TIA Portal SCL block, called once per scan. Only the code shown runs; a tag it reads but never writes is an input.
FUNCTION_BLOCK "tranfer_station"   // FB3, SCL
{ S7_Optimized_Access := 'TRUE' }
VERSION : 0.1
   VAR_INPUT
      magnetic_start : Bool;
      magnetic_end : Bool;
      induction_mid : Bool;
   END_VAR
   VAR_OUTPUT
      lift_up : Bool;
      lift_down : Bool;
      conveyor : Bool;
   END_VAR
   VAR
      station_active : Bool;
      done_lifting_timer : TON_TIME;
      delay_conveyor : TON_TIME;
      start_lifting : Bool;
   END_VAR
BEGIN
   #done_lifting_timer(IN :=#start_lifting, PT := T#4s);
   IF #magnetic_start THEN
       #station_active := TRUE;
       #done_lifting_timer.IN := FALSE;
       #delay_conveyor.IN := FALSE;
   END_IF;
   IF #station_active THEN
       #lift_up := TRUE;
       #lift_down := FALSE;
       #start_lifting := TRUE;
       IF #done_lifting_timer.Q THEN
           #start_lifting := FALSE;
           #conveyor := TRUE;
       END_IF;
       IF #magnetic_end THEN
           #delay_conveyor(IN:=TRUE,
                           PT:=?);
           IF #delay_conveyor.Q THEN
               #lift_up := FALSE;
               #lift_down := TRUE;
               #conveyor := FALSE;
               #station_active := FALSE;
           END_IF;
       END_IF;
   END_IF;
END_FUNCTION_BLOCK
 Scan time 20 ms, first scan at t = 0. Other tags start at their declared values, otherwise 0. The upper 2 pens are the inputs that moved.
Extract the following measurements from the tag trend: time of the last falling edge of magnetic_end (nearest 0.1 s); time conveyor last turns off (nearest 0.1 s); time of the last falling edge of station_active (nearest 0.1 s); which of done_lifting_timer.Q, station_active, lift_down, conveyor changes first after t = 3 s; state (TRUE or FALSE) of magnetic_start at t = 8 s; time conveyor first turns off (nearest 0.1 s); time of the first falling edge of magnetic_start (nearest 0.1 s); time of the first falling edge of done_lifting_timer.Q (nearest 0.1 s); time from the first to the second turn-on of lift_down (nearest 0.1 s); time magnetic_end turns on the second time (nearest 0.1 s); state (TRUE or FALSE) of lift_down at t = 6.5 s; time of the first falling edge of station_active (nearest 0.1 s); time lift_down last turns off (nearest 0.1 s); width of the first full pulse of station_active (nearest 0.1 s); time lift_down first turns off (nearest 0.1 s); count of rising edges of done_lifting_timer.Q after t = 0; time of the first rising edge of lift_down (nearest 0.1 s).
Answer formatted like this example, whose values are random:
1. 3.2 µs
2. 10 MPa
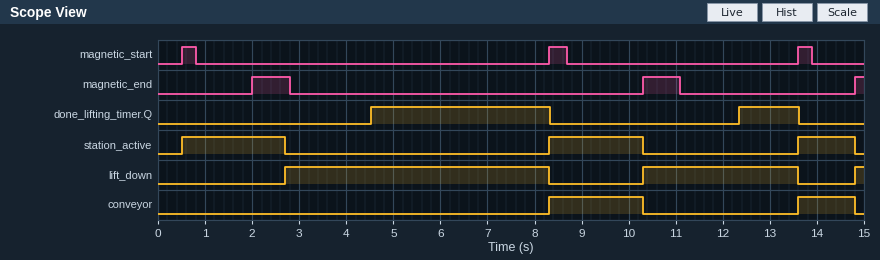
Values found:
1. 11.1 s
2. 14.8 s
3. 14.8 s
4. done_lifting_timer.Q
5. FALSE
6. 10.3 s
7. 0.8 s
8. 8.3 s
9. 7.6 s
10. 10.3 s
11. TRUE
12. 2.7 s
13. 13.6 s
14. 2.2 s
15. 8.3 s
16. 2
17. 2.7 s
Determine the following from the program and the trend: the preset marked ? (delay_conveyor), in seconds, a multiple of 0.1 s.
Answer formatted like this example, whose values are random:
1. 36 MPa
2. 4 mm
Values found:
1. 0.7 s
